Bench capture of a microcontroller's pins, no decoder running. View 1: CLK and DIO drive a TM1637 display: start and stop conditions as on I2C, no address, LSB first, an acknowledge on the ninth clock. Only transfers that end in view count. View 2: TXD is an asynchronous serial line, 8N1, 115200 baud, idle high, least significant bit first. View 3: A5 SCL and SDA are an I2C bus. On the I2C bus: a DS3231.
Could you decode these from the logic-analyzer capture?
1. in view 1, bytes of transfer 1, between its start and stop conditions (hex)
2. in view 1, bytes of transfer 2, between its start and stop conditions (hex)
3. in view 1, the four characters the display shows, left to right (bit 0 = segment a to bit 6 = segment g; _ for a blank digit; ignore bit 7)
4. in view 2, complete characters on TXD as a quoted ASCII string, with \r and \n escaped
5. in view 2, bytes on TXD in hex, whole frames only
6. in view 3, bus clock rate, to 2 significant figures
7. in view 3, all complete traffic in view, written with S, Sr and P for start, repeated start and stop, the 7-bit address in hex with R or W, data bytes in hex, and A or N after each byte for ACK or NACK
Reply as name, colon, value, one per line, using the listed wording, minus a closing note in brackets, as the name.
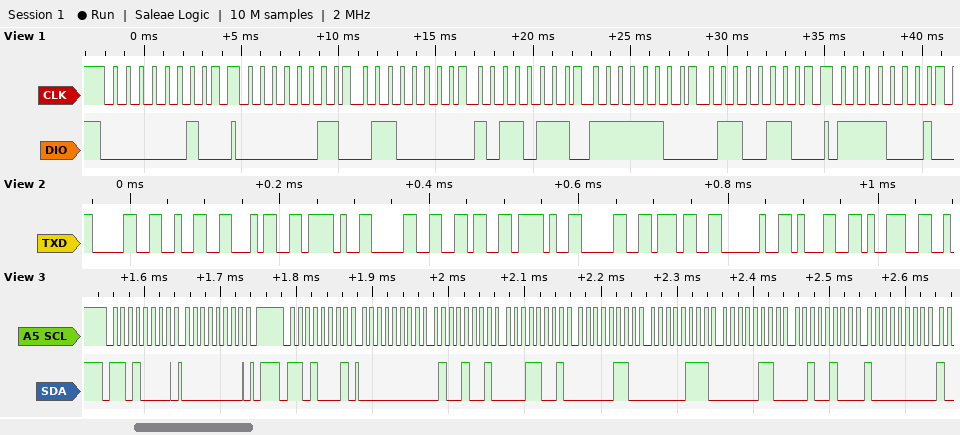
in view 1, bytes of transfer 1, between its start and stop conditions: 40
in view 1, bytes of transfer 2, between its start and stop conditions: C0 06 ED 3F 66
in view 1, the four characters the display shows, left to right: 1504
in view 2, complete characters on TXD as a quoted ASCII string, with \r and \n escaped: "024/06/07 19"
in view 2, bytes on TXD in hex, whole frames only: 30 32 34 2F 30 36 2F 30 37 20 31 39
in view 3, bus clock rate, to 2 significant figures: 100 kHz
in view 3, all complete traffic in view, written with S, Sr and P for start, repeated start and stop, the 7-bit address in hex with R or W, data bytes in hex, and A or N after each byte for ACK or NACK: S 68W A 00 A P S 68R A 00 A 49 A 19 A 06 A 07 A 06 A 24 A 80 A
